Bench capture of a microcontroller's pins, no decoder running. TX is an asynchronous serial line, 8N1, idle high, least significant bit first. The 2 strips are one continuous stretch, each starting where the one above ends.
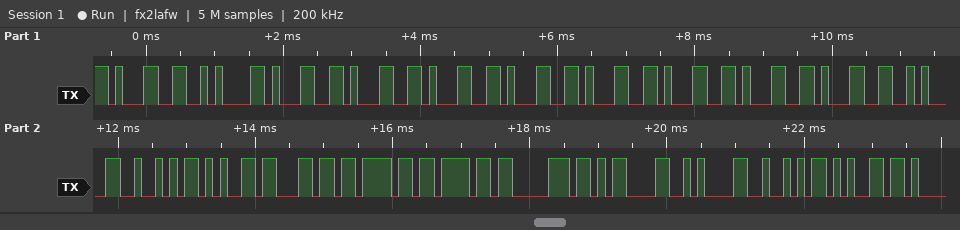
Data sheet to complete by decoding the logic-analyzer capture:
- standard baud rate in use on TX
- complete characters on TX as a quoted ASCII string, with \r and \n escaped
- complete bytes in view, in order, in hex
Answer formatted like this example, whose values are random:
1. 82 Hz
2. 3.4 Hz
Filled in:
1. 9600 baud
2. "1\n11111111\nReloop\r\nRe"
3. 0x31 0x0A 0x31 0x31 0x31 0x31 0x31 0x31 0x31 0x31 0x0A 0x52 0x65 0x6C 0x6F 0x6F 0x70 0x0D 0x0A 0x52 0x65
